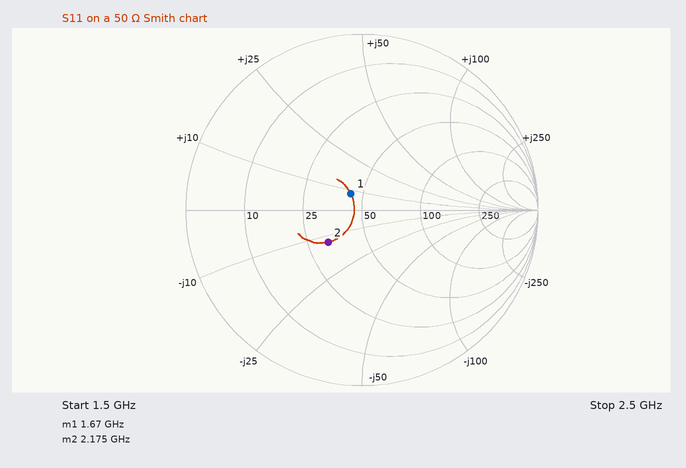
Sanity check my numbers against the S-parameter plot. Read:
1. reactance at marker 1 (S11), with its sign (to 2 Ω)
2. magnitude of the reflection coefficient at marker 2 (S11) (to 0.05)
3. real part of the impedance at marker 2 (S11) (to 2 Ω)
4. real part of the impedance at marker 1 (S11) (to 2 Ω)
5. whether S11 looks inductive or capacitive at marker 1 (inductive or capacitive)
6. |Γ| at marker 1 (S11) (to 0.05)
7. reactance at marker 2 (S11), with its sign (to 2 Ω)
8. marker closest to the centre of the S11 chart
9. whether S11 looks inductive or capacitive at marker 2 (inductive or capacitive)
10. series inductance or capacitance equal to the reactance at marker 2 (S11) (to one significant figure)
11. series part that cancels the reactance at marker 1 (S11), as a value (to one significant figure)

+8 Ω
0.25
32 Ω
44 Ω
inductive
0.10
-12 Ω
marker 1
capacitive
6 pF
10 pF
